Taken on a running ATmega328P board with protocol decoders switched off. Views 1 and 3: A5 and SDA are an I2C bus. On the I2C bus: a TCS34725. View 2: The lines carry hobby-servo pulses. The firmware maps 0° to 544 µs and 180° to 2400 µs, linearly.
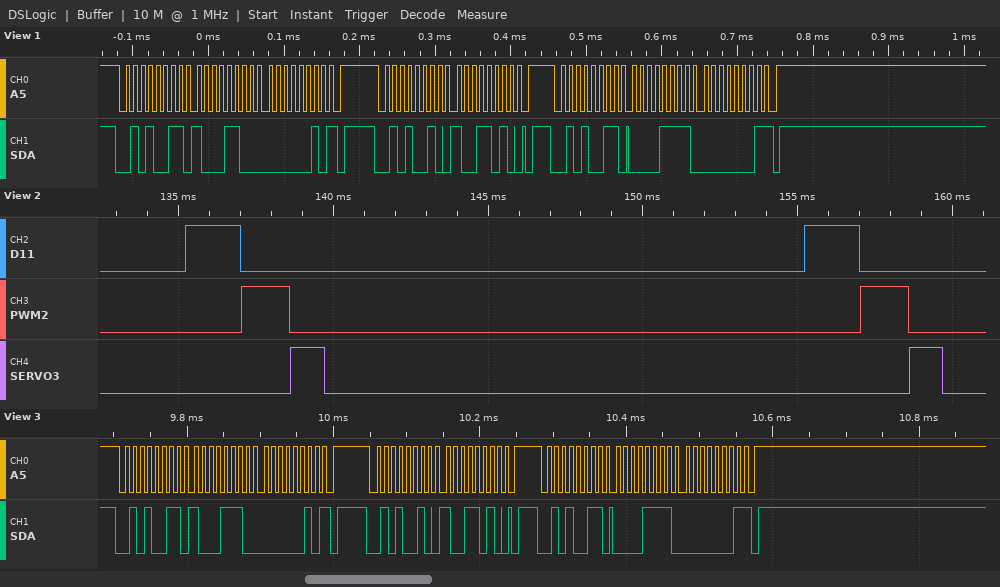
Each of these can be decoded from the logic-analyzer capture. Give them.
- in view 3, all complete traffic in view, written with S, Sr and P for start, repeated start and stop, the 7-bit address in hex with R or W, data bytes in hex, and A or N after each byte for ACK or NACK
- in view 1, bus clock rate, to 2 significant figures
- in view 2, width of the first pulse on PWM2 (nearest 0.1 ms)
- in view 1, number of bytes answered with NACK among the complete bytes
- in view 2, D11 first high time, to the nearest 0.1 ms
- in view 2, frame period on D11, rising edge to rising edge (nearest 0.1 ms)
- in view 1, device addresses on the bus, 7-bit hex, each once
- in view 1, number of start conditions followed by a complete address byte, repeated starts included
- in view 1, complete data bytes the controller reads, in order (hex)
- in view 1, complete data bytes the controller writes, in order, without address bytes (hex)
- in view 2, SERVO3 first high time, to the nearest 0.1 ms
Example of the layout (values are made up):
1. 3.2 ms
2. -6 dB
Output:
1. S 29R A 8E A 02 N P S 29W A 9A A P S 29R A 0F A 01 N P
2. 100 kHz
3. 1.6 ms
4. 2
5. 1.8 ms
6. 20.0 ms
7. 0x29
8. 3
9. 8C 02 0F 01
10. 9A
11. 1.1 ms
